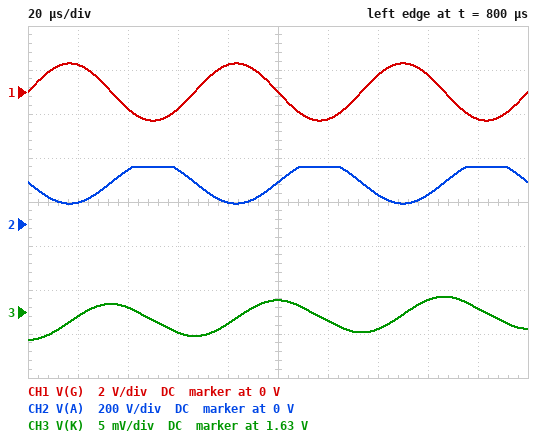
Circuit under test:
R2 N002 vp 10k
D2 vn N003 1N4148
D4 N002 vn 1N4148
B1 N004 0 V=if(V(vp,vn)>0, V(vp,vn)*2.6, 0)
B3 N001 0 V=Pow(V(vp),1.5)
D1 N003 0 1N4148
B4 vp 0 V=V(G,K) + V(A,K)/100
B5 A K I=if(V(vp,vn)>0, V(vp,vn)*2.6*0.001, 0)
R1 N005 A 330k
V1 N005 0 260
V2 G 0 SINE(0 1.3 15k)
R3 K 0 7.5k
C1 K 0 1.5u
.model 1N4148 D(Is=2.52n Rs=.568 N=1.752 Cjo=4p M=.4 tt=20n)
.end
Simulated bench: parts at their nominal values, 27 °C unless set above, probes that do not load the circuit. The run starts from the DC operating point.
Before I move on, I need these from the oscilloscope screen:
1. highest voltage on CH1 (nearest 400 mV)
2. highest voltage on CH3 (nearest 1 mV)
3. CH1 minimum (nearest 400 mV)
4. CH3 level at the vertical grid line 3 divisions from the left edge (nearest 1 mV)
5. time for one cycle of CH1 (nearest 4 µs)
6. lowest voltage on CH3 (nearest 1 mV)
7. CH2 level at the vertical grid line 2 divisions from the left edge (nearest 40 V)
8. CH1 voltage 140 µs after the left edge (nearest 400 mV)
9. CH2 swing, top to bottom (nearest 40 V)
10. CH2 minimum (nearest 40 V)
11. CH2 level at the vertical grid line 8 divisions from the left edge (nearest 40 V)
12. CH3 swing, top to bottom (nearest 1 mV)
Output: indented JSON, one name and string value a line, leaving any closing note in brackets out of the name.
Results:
{
  "highest voltage on CH1": "1.2 V",
  "highest voltage on CH3": "1.632 V",
  "CH1 minimum": "-1.2 V",
  "CH3 level at the vertical grid line 3 divisions from the left edge": "1.628 V",
  "time for one cycle of CH1": "68 µs",
  "lowest voltage on CH3": "1.627 V",
  "CH2 level at the vertical grid line 2 divisions from the left edge": "240 V",
  "CH1 voltage 140 µs after the left edge": "800 mV",
  "CH2 swing, top to bottom": "160 V",
  "CH2 minimum": "80 V",
  "CH2 level at the vertical grid line 8 divisions from the left edge": "120 V",
  "CH3 swing, top to bottom": "5 mV"
}
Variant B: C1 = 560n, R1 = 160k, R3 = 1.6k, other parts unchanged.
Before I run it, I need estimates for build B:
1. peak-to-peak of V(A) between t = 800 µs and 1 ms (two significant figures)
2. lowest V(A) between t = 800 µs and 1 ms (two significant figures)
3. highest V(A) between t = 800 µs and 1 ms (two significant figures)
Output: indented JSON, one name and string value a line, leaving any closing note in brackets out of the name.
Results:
{
  "peak-to-peak of V(A) between t = 800 µs and 1 ms": "160 V",
  "lowest V(A) between t = 800 µs and 1 ms": "82 V",
  "highest V(A) between t = 800 µs and 1 ms": "240 V"
}
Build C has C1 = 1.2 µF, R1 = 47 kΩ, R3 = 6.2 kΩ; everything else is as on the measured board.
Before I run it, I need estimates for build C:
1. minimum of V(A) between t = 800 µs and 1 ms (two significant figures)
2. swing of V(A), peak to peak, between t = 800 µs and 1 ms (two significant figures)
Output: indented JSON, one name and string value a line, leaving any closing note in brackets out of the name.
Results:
{
  "minimum of V(A) between t = 800 µs and 1 ms": "200 V",
  "swing of V(A), peak to peak, between t = 800 µs and 1 ms": "56 V"
}
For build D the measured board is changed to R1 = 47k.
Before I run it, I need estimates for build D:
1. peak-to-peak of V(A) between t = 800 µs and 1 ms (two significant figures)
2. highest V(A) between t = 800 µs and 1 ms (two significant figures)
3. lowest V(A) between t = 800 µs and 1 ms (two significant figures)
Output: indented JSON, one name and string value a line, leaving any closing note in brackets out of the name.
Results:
{
  "peak-to-peak of V(A) between t = 800 µs and 1 ms": "53 V",
  "highest V(A) between t = 800 µs and 1 ms": "260 V",
  "lowest V(A) between t = 800 µs and 1 ms": "210 V"
}
